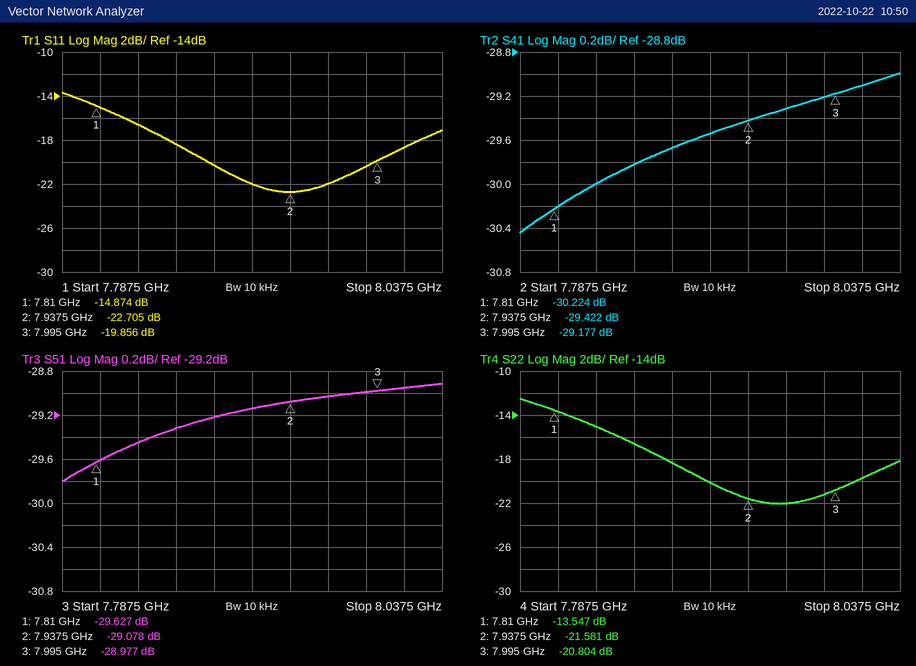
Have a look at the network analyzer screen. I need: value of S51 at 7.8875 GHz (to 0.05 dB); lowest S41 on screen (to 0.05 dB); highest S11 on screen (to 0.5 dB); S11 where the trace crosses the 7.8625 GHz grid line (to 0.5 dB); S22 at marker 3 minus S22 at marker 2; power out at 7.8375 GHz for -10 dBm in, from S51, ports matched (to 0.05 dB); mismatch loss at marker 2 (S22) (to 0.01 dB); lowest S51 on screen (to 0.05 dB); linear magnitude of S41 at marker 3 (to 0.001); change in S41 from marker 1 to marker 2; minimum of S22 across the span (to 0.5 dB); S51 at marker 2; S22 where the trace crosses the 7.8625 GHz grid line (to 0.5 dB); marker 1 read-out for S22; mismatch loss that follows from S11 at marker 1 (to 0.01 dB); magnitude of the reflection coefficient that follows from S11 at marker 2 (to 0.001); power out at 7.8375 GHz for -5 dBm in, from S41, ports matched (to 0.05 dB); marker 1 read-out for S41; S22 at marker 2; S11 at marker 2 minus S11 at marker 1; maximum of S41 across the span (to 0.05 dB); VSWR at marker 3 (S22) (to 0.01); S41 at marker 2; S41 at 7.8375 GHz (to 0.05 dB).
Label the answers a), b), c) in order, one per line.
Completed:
a) -29.20 dB
b) -30.45 dB
c) -13.5 dB
d) -18.5 dB
e) 0.777 dB
f) -39.45 dBm
g) 0.03 dB
h) -29.80 dB
i) 0.035
j) 0.802 dB
k) -22.0 dB
l) -29.078 dB
m) -16.5 dB
n) -13.547 dB
o) 0.14 dB
p) 0.073
q) -35.00 dBm
r) -30.224 dB
s) -21.581 dB
t) -7.831 dB
u) -29.00 dB
v) 1.20
w) -29.422 dB
x) -30.00 dB
